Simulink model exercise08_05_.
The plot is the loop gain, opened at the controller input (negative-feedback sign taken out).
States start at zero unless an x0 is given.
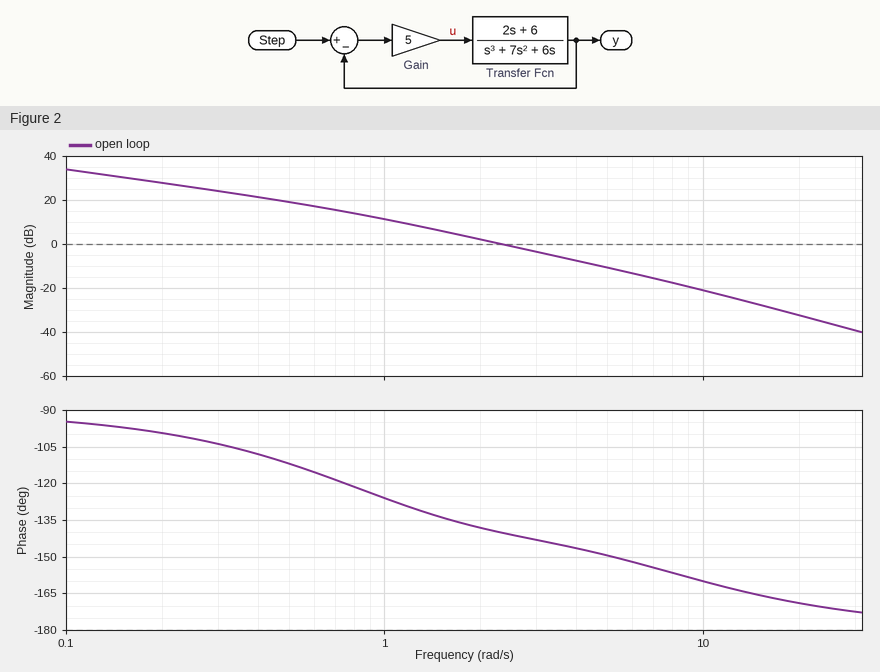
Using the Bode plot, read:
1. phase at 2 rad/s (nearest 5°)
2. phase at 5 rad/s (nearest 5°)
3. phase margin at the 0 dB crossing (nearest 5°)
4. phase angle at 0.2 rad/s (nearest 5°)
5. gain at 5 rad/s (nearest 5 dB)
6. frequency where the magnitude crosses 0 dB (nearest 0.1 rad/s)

-140°
-150°
40°
-100°
-10 dB
2.3 rad/s
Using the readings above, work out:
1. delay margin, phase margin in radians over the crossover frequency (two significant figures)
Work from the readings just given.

0.30 s
